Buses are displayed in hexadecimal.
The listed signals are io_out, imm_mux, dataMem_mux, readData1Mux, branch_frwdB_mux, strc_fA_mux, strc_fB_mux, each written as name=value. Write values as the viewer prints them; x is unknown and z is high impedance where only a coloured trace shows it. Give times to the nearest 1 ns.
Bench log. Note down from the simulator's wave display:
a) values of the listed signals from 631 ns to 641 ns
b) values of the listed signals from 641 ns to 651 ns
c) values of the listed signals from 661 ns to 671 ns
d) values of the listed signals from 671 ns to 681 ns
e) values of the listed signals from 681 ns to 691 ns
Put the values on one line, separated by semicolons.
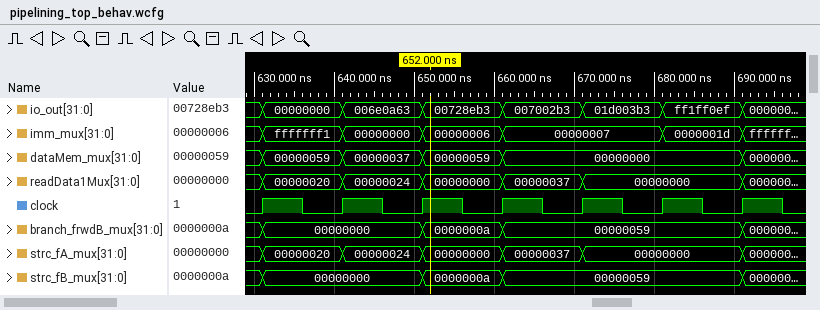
io_out=00000000, imm_mux=fffffff1, dataMem_mux=00000059, readData1Mux=00000020, branch_frwdB_mux=00000000, strc_fA_mux=00000020, strc_fB_mux=00000000; io_out=006e0a63, imm_mux=00000000, dataMem_mux=00000037, readData1Mux=00000024, branch_frwdB_mux=00000000, strc_fA_mux=00000024, strc_fB_mux=00000000; io_out=007002b3, imm_mux=00000007, dataMem_mux=00000000, readData1Mux=00000037, branch_frwdB_mux=00000059, strc_fA_mux=00000037, strc_fB_mux=00000059; io_out=01d003b3, imm_mux=00000007, dataMem_mux=00000000, readData1Mux=00000000, branch_frwdB_mux=00000059, strc_fA_mux=00000000, strc_fB_mux=00000059; io_out=ff1ff0ef, imm_mux=0000001d, dataMem_mux=00000000, readData1Mux=00000000, branch_frwdB_mux=00000059, strc_fA_mux=00000000, strc_fB_mux=00000059
